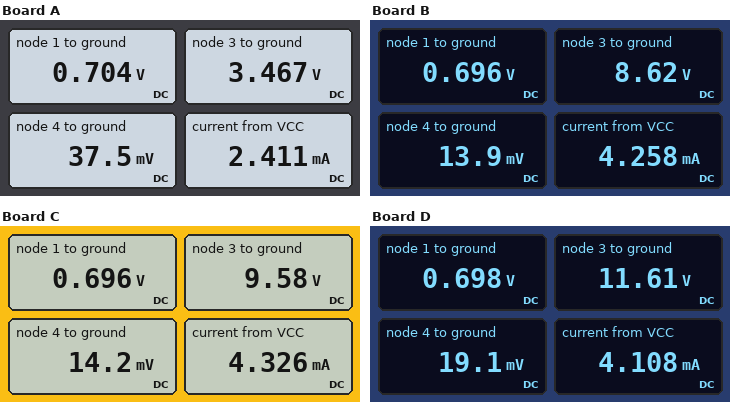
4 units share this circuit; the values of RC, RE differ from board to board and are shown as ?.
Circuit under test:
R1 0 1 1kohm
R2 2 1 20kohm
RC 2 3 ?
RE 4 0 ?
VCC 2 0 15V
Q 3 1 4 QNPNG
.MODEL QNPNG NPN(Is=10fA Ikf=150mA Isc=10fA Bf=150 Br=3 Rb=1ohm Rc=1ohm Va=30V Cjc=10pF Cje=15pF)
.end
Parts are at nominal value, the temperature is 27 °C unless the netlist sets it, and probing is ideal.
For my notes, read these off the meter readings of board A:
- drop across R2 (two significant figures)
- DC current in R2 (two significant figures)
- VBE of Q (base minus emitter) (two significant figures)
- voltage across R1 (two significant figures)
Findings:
14 V
710 µA
670 mV
700 mV
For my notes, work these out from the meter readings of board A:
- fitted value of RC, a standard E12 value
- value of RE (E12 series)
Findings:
6.8 kΩ
22 Ω
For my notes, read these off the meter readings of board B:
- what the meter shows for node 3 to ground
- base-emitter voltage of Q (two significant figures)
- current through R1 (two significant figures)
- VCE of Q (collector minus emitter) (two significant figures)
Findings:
8.62 V
680 mV
700 µA
8.6 V
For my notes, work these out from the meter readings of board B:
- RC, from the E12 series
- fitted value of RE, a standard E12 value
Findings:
1.8 kΩ
3.9 Ω
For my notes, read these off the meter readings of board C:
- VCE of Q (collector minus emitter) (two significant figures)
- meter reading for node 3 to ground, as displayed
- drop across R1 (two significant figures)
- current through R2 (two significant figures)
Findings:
9.6 V
9.58 V
700 mV
720 µA
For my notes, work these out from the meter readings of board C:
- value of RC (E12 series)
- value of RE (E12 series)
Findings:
1.5 kΩ
3.9 Ω
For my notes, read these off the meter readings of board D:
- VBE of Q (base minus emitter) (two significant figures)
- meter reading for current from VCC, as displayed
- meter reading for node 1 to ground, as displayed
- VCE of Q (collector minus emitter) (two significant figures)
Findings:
680 mV
4.108 mA
0.698 V
12 V
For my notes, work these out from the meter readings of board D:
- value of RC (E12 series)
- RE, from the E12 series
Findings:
1 kΩ
5.6 Ω
